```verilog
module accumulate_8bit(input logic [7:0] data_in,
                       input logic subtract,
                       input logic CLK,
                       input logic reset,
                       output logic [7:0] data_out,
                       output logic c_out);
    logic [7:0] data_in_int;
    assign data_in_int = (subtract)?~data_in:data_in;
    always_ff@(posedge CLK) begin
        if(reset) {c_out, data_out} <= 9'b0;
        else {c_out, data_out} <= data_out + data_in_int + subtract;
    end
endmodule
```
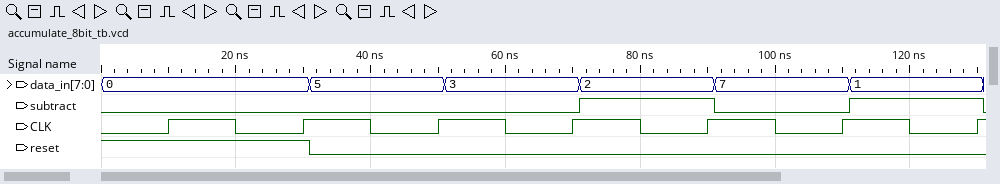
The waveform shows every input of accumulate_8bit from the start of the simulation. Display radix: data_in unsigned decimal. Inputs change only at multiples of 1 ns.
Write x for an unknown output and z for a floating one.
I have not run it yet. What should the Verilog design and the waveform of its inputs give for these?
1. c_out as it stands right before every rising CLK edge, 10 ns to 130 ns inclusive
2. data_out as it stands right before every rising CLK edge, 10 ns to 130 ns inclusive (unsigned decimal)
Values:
x 0 0 0 0 1 0
x, 0, 0, 5, 8, 6, 13
